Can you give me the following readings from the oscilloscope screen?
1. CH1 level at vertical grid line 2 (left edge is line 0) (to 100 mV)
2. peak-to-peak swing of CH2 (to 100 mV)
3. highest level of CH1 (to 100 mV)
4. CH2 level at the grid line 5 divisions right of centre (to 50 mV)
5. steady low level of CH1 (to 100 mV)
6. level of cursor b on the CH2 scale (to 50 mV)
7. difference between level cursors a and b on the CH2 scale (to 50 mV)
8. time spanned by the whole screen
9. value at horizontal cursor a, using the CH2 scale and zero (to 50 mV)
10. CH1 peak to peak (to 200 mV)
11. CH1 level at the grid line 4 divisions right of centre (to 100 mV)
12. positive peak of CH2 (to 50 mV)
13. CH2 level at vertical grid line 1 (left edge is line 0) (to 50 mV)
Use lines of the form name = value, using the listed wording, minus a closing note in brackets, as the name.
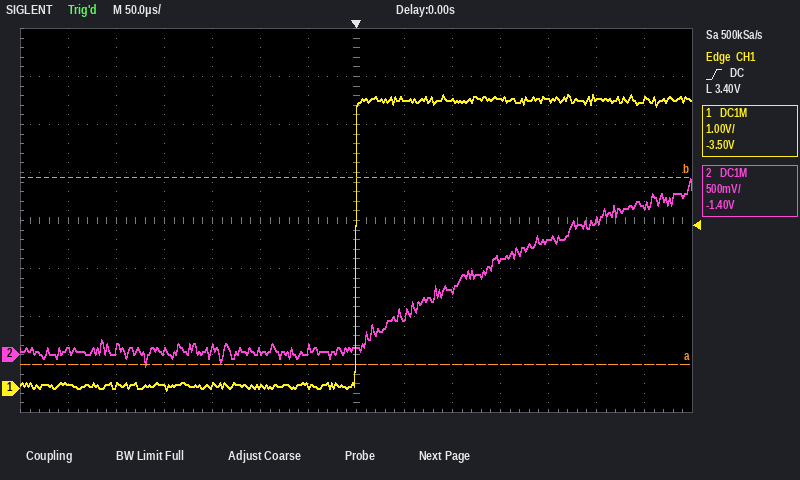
CH1 level at vertical grid line 2 (left edge is line 0) = 100 mV
peak-to-peak swing of CH2 = 2.00 V
highest level of CH1 = 6.1 V
CH2 level at the grid line 5 divisions right of centre = 1.40 V
steady low level of CH1 = 100 mV
level of cursor b on the CH2 scale = 1.85 V
difference between level cursors a and b on the CH2 scale = 1.95 V
time spanned by the whole screen = 700 µs
value at horizontal cursor a, using the CH2 scale and zero = -100 mV
CH1 peak to peak = 6.2 V
CH1 level at the grid line 4 divisions right of centre = 6.0 V
positive peak of CH2 = 1.85 V
CH2 level at vertical grid line 1 (left edge is line 0) = 50 mV
